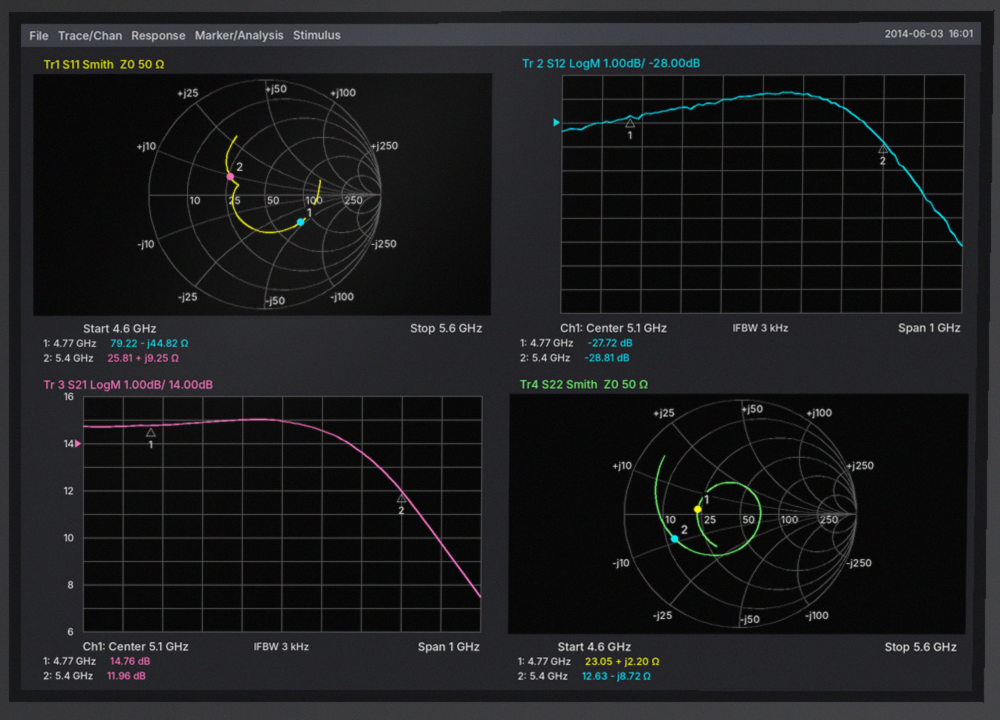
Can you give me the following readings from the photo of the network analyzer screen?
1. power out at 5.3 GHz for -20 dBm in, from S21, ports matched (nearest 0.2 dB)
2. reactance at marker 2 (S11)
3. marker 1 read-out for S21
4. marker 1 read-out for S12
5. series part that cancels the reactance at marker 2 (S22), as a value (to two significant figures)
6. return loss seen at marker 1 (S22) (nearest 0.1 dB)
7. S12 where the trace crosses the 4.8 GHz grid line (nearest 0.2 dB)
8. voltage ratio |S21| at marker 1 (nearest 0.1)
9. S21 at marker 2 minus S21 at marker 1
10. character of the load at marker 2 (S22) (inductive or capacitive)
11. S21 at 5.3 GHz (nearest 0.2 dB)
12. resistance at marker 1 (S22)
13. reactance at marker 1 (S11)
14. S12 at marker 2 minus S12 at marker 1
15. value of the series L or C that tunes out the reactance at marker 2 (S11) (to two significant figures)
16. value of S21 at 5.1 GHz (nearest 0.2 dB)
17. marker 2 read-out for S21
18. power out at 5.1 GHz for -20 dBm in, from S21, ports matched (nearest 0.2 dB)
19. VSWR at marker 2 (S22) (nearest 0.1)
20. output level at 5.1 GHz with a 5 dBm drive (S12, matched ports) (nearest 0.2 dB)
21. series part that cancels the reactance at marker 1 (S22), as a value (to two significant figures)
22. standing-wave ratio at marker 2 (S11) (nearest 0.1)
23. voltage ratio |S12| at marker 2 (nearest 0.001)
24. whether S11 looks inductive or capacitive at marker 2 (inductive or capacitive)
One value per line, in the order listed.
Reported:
-6.4 dBm
+9.25 Ω
14.76 dB
-27.72 dB
260 pH
8.6 dB
-27.6 dB
5.5
-2.80 dB
capacitive
13.6 dB
23.05 Ω
-44.82 Ω
-1.09 dB
3.2 pF
15.0 dB
11.96 dB
-5.0 dBm
4.1
-21.8 dBm
15 pF
2.0
0.036
inductive
